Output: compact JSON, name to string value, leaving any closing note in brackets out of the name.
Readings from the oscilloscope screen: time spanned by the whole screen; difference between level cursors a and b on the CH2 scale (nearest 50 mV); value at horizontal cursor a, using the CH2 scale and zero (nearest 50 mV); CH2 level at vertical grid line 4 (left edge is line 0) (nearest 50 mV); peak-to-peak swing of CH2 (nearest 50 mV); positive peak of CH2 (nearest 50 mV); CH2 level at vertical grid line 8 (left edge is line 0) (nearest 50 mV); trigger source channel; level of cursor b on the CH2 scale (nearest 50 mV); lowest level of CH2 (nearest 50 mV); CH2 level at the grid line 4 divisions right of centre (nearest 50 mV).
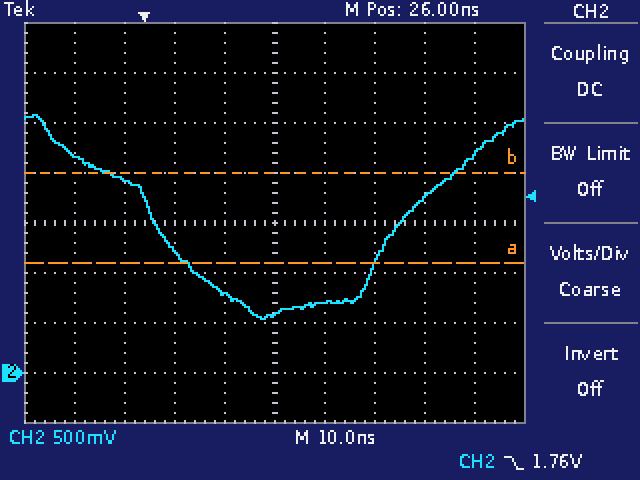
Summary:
{"time spanned by the whole screen": "100 ns", "difference between level cursors a and b on the CH2 scale": "900 mV", "value at horizontal cursor a, using the CH2 scale and zero": "1.10 V", "CH2 level at vertical grid line 4 (left edge is line 0)": "800 mV", "peak-to-peak swing of CH2": "2.05 V", "positive peak of CH2": "2.60 V", "CH2 level at vertical grid line 8 (left edge is line 0)": "1.75 V", "trigger source channel": "CH2", "level of cursor b on the CH2 scale": "2.00 V", "lowest level of CH2": "550 mV", "CH2 level at the grid line 4 divisions right of centre": "2.20 V"}
